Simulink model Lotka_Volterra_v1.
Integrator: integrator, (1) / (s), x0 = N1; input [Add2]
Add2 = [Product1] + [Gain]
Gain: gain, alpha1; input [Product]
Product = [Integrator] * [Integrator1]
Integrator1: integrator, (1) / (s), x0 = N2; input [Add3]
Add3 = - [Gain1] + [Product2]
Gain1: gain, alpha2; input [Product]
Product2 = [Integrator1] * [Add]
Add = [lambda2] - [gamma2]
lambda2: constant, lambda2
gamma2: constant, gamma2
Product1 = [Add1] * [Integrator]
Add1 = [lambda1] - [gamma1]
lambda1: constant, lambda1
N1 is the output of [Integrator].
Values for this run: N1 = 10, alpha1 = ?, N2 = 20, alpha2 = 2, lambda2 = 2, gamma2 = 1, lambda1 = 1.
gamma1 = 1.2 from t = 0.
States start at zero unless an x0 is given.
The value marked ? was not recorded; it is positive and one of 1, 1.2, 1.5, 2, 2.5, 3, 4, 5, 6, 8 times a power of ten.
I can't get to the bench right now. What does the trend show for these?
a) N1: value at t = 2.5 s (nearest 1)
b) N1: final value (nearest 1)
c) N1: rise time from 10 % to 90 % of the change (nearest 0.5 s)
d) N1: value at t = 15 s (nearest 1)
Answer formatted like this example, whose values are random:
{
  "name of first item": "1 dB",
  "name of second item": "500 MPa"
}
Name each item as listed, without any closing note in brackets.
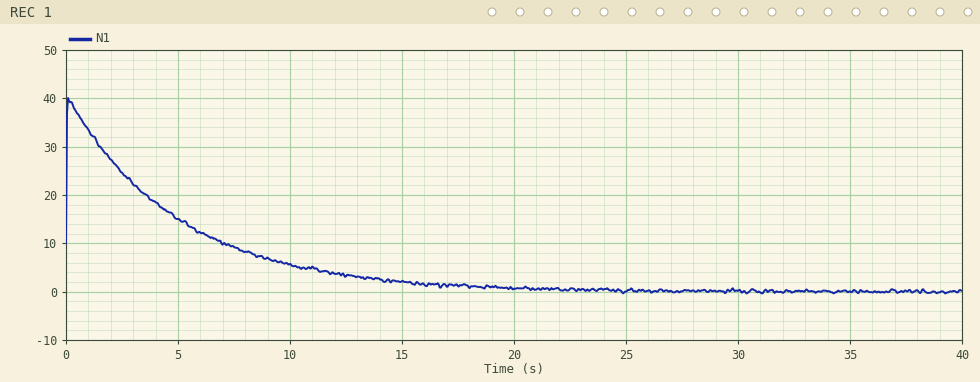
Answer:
{
  "N1: value at t = 2.5 s": "25",
  "N1: final value": "0",
  "N1: rise time from 10 % to 90 % of the change": "11.0 s",
  "N1: value at t = 15 s": "2"
}
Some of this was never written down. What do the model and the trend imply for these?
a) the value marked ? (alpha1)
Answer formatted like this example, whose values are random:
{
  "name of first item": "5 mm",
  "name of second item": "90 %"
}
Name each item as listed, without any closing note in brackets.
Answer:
{
  "the value marked ?": "3"
}
